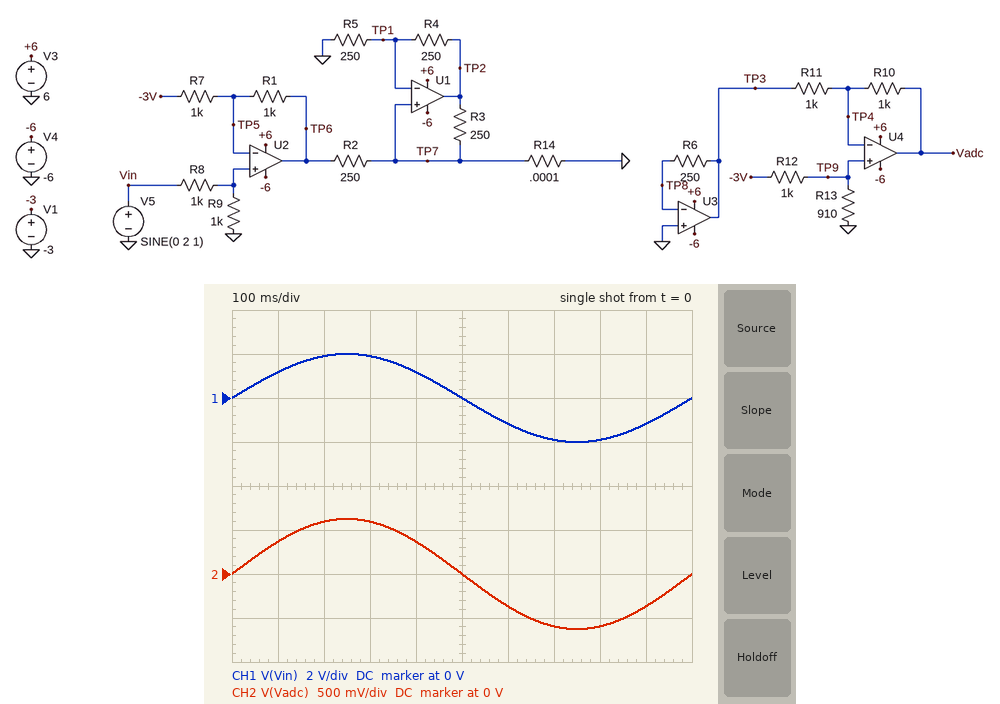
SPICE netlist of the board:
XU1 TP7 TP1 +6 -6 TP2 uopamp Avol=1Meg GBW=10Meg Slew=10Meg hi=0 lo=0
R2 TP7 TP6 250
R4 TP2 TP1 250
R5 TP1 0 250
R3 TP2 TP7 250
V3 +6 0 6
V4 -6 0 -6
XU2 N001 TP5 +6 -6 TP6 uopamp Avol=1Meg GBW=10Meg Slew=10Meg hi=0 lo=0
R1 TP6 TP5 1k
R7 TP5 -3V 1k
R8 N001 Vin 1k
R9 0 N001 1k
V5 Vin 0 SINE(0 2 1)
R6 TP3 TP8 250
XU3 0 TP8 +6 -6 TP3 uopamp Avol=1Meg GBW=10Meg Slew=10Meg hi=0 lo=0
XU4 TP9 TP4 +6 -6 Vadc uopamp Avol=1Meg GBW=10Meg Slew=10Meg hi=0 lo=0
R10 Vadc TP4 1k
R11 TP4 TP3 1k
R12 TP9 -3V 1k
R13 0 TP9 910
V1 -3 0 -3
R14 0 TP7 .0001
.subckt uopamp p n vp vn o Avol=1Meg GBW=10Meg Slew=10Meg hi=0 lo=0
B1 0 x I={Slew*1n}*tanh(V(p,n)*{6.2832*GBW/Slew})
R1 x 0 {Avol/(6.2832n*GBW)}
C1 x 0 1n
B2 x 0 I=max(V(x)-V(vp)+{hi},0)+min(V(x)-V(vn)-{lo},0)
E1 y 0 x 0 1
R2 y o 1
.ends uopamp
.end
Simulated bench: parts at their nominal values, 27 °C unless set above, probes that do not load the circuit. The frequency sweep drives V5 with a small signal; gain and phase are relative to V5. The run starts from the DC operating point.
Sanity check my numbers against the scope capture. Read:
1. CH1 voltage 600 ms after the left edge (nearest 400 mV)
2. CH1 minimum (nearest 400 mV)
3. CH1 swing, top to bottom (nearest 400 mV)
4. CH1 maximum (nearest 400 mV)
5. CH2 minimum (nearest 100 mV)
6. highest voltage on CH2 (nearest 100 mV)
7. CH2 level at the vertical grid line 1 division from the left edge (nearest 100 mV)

-1.2 V
-2.0 V
4.0 V
2.0 V
-600 mV
600 mV
400 mV
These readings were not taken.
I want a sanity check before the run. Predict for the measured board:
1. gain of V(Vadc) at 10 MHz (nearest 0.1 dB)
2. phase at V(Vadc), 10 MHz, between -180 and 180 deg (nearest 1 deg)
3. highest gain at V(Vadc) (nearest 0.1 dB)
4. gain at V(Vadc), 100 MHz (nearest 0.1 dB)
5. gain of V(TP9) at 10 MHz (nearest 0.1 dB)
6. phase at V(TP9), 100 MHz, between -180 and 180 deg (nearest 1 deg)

-21.6 dB
-117 deg
-10.1 dB
-58.8 dB
-20.6 dB
-86 deg
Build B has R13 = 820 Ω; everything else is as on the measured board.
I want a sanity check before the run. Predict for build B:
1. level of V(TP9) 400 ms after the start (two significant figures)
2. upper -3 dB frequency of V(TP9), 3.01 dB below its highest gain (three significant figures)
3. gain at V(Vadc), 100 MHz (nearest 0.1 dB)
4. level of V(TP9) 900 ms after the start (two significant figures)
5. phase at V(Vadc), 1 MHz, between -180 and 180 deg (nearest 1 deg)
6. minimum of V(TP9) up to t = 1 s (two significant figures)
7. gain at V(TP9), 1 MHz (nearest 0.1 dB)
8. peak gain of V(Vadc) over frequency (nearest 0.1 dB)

170 mV
7.35 MHz
-59.5 dB
-170 mV
-19 deg
-290 mV
-16.8 dB
-10.7 dB
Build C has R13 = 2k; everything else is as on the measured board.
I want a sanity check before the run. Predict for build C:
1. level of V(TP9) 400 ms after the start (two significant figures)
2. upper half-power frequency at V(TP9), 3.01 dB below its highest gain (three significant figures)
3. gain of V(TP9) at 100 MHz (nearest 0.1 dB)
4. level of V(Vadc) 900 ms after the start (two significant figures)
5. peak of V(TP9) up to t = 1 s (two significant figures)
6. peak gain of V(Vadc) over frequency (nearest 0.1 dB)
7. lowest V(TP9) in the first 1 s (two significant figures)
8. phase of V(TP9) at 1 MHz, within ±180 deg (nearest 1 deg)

290 mV
7.97 MHz
-34.0 dB
-590 mV
500 mV
-6.0 dB
-500 mV
-7 deg
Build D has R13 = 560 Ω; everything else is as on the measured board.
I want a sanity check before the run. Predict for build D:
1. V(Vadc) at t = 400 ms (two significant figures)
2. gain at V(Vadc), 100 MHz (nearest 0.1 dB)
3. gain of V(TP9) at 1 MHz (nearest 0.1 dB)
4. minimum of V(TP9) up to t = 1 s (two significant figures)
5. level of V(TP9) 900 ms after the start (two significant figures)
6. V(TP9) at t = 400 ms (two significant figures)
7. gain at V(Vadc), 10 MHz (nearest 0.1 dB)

260 mV
-62.2 dB
-19.3 dB
-220 mV
-130 mV
130 mV
-24.9 dB
